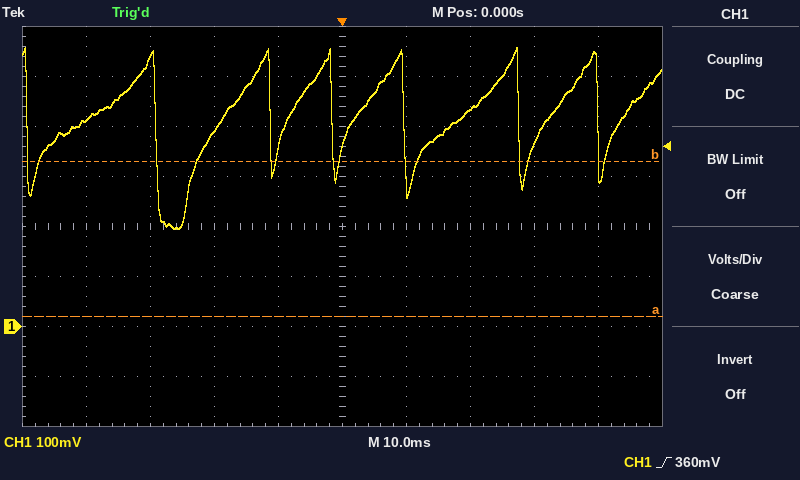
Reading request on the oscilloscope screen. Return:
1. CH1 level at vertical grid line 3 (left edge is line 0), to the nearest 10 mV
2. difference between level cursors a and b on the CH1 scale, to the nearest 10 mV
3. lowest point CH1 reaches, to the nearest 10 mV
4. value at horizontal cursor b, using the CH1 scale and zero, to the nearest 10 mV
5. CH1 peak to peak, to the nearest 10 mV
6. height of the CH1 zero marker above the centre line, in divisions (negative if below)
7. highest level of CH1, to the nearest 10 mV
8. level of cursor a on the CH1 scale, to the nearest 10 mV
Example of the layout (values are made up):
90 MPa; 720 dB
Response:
390 mV; 310 mV; 200 mV; 330 mV; 360 mV; -2.0 div; 560 mV; 20 mV
